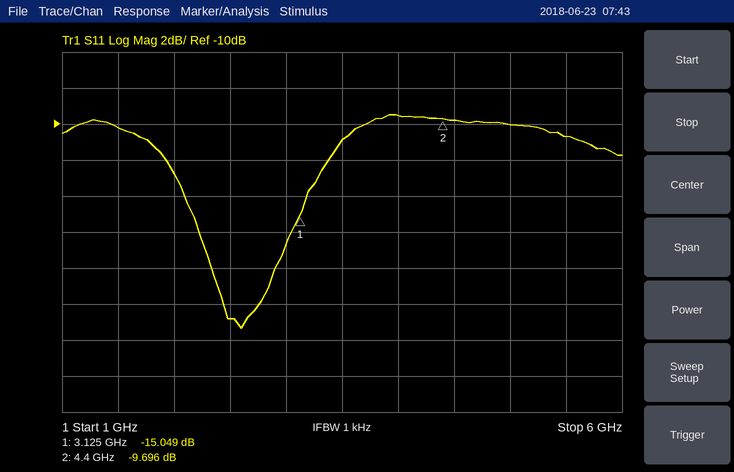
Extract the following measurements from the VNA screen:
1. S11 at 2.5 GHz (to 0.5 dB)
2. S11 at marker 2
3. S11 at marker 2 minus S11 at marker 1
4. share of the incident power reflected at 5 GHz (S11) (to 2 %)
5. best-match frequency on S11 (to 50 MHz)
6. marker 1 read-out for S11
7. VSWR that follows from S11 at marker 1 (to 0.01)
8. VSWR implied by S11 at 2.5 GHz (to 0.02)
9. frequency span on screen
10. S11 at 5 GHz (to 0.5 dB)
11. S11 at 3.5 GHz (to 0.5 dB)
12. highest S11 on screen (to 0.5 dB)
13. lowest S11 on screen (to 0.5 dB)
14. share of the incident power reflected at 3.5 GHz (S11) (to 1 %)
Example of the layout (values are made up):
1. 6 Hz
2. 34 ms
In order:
1. -21.0 dB
2. -9.696 dB
3. 5.353 dB
4. 10 %
5. 2.60 GHz
6. -15.049 dB
7. 1.43
8. 1.20
9. 5 GHz
10. -10.0 dB
11. -11.0 dB
12. -9.5 dB
13. -21.5 dB
14. 8 %
